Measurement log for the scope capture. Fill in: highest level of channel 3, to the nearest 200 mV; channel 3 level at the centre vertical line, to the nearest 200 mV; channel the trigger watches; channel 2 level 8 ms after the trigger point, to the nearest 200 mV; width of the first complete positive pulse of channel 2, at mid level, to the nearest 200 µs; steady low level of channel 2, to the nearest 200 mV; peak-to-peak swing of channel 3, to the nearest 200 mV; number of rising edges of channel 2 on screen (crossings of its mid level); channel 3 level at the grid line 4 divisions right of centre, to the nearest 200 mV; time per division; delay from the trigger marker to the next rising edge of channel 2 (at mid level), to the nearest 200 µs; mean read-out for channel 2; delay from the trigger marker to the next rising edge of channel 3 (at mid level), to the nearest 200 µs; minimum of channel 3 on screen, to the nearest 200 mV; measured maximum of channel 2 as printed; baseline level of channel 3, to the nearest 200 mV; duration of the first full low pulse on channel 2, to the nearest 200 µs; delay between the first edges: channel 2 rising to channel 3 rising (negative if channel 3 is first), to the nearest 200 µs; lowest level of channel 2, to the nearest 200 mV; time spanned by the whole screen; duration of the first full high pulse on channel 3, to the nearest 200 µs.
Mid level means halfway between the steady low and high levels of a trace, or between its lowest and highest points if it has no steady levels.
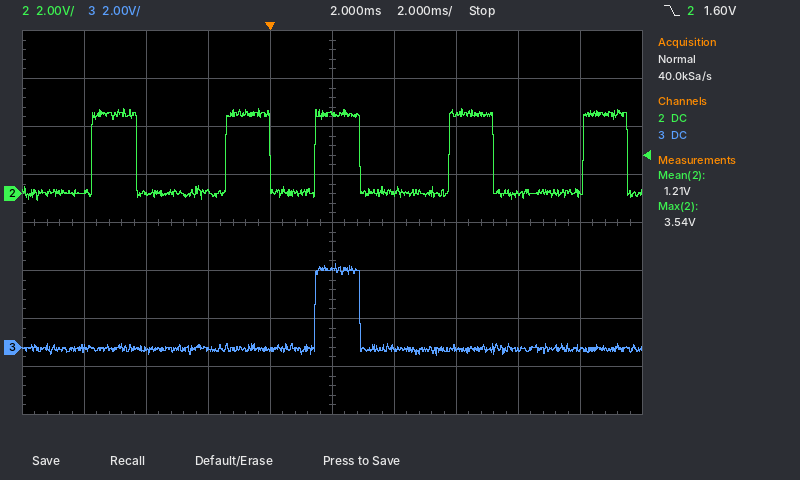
3.4 V
3.2 V
channel 2
0.0 V
1.4 ms
0.0 V
3.8 V
5
0.0 V
2 ms
1.4 ms
1.21 V
1.4 ms
-400 mV
3.54 V
0.0 V
2.8 ms
+7.2 ms
-200 mV
20 ms
1.4 ms
